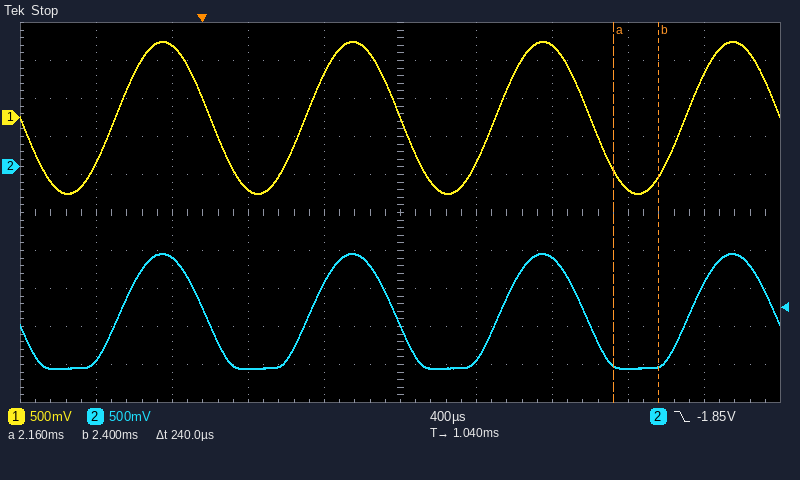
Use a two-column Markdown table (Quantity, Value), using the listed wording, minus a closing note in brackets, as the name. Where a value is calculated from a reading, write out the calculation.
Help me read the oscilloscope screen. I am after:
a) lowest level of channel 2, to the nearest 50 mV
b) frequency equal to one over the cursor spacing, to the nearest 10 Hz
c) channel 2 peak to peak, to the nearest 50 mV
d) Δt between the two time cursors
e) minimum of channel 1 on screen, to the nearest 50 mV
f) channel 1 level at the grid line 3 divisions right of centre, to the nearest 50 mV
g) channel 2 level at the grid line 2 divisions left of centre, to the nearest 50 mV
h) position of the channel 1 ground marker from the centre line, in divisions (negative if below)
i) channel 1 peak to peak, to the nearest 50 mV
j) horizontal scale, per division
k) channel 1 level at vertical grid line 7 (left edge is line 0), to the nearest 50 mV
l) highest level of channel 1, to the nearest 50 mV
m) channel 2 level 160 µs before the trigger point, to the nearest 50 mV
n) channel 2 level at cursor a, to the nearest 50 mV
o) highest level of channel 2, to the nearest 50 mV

| Quantity | Value |
|---|---|
| lowest level of channel 2, to the nearest 50 mV | -2.65 V |
| frequency equal to one over the cursor spacing, to the nearest 10 Hz | 1 / 240 µs ≈ 4.17 kHz |
| channel 2 peak to peak, to the nearest 50 mV | -1.15 V − (-2.65 V) = 1.50 V |
| Δt between the two time cursors | 240 µs |
| minimum of channel 1 on screen, to the nearest 50 mV | -1.00 V |
| channel 1 level at the grid line 3 divisions right of centre, to the nearest 50 mV | -950 mV |
| channel 2 level at the grid line 2 divisions left of centre, to the nearest 50 mV | -2.65 V |
| position of the channel 1 ground marker from the centre line, in divisions | +2.5 div |
| channel 1 peak to peak, to the nearest 50 mV | 1.00 V − (-1.00 V) = 2.00 V |
| horizontal scale, per division | 400 µs |
| channel 1 level at vertical grid line 7 (left edge is line 0), to the nearest 50 mV | 950 mV |
| highest level of channel 1, to the nearest 50 mV | 1.00 V |
| channel 2 level 160 µs before the trigger point, to the nearest 50 mV | -1.20 V |
| channel 2 level at cursor a, to the nearest 50 mV | -2.60 V |
| highest level of channel 2, to the nearest 50 mV | -1.15 V |
